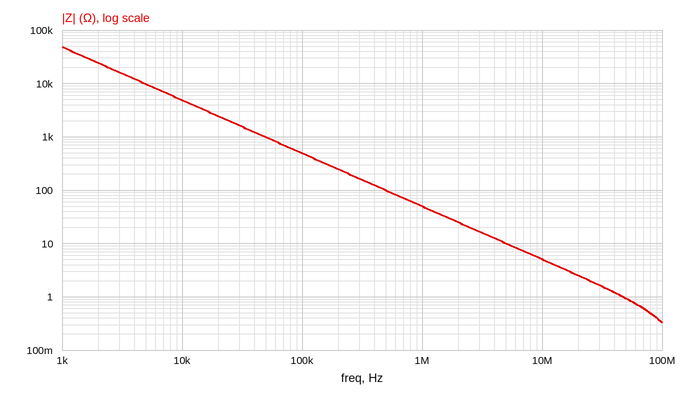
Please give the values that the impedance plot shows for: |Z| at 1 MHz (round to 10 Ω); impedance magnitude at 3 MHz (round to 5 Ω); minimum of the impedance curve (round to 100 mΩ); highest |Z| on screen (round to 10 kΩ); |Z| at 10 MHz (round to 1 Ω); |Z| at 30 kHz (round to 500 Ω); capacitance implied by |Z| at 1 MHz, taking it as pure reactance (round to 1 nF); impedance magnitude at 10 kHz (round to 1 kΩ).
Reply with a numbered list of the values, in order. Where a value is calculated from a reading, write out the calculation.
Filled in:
1. 50 Ω
2. 15 Ω
3. 300 mΩ
4. 50 kΩ
5. 5 Ω
6. 1.5 kΩ
7. C = 1/(2π × 1 MHz × 50 Ω) ≈ 3 nF
8. 5 kΩ
